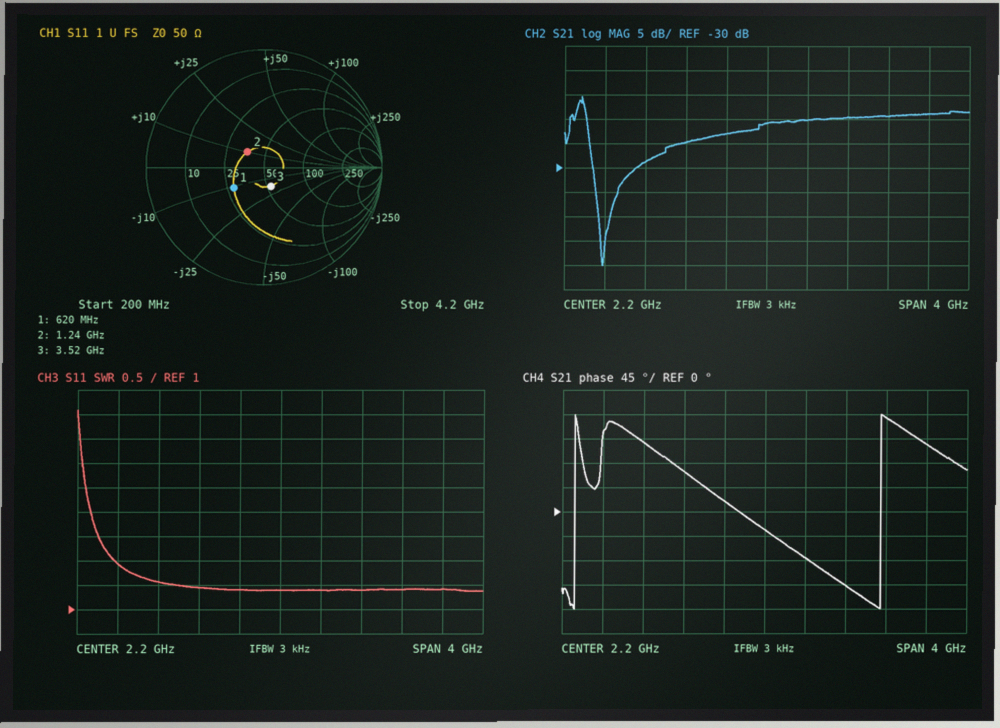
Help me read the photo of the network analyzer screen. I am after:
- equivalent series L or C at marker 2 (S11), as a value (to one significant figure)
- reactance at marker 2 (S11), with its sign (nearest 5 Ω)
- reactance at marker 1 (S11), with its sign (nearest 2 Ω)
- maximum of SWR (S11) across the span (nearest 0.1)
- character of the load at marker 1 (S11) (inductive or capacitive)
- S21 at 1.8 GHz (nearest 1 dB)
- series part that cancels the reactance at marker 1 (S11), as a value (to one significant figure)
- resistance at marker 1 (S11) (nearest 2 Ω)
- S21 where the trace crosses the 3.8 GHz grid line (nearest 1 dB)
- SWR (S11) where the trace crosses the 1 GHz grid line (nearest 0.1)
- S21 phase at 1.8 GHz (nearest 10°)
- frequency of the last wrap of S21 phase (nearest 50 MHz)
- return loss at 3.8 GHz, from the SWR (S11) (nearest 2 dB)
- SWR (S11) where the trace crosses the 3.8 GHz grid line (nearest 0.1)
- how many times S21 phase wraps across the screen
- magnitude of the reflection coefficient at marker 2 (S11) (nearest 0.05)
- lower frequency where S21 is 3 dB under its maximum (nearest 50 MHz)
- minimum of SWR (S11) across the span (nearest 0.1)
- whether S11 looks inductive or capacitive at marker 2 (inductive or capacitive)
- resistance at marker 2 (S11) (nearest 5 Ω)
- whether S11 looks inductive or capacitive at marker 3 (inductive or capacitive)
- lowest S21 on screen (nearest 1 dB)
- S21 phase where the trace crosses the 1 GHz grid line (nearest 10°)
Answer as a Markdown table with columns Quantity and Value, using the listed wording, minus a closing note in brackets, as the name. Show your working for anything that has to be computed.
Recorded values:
| Quantity | Value |
|---|---|
| equivalent series L or C at marker 2 (S11), as a value | L = 10 Ω/(2π × 1.24 GHz) ≈ 1 nH |
| reactance at marker 2 (S11), with its sign | +10 Ω |
| reactance at marker 1 (S11), with its sign | -10 Ω |
| maximum of SWR (S11) across the span | 5.1 |
| character of the load at marker 1 (S11) | capacitive |
| S21 at 1.8 GHz | -23 dB |
| series part that cancels the reactance at marker 1 (S11), as a value | L = 10 Ω/(2π × 620 MHz) ≈ 3 nH |
| resistance at marker 1 (S11) | 28 Ω |
| S21 where the trace crosses the 3.8 GHz grid line | -19 dB |
| SWR (S11) where the trace crosses the 1 GHz grid line | 1.6 |
| S21 phase at 1.8 GHz | 20° |
| frequency of the last wrap of S21 phase | 3.35 GHz |
| return loss at 3.8 GHz, from the SWR (S11) | −20 log10((1.4 − 1)/(1.4 + 1)) ≈ 16 dB |
| SWR (S11) where the trace crosses the 3.8 GHz grid line | 1.4 |
| how many times S21 phase wraps across the screen | 2 |
| magnitude of the reflection coefficient at marker 2 (S11) | 0.20 |
| lower frequency where S21 is 3 dB under its maximum | 300 MHz |
| minimum of SWR (S11) across the span | 1.4 |
| whether S11 looks inductive or capacitive at marker 2 | inductive |
| resistance at marker 2 (S11) | 35 Ω |
| whether S11 looks inductive or capacitive at marker 3 | capacitive |
| lowest S21 on screen | -50 dB |
| S21 phase where the trace crosses the 1 GHz grid line | 130° |
